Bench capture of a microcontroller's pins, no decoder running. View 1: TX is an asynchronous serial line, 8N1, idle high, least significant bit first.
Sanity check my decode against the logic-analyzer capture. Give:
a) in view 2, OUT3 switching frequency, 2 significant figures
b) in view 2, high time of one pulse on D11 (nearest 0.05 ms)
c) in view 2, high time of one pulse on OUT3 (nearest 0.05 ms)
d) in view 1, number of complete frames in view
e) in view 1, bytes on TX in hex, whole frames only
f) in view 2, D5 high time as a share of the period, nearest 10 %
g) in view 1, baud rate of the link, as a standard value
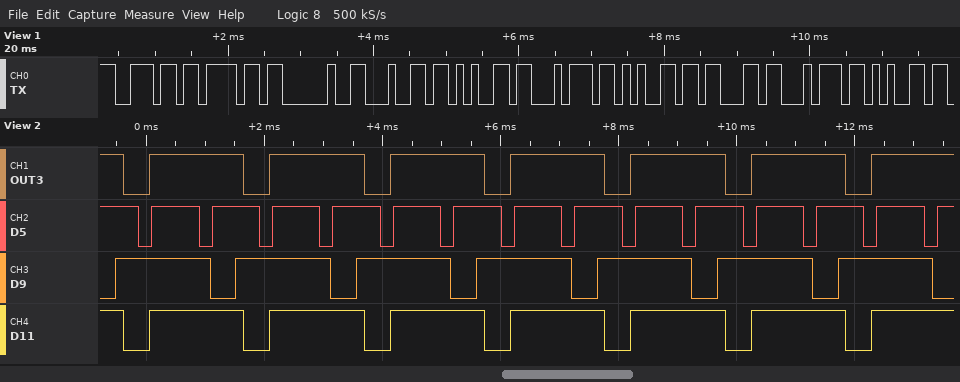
490 Hz
1.60 ms
1.60 ms
10
6E 6F 20 64 65 74 65 63 74 65
80 %
9600 baud
